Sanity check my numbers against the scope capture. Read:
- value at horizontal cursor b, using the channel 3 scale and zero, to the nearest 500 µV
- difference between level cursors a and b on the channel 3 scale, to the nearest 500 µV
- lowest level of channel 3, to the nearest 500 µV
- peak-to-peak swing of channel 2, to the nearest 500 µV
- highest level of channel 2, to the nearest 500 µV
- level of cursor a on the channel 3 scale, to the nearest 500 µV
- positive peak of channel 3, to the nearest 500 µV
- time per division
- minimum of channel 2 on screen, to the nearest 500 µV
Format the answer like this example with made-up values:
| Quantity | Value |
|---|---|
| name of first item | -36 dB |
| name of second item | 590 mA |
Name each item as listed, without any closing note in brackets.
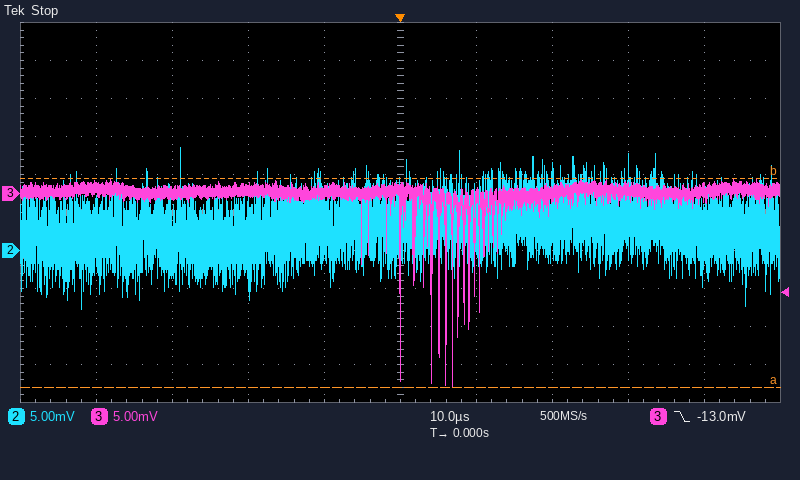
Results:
| Quantity | Value |
|---|---|
| value at horizontal cursor b, using the channel 3 scale and zero, to the nearest 500 µV | 2.0 mV |
| difference between level cursors a and b on the channel 3 scale, to the nearest 500 µV | 27.5 mV |
| lowest level of channel 3, to the nearest 500 µV | -25.5 mV |
| peak-to-peak swing of channel 2, to the nearest 500 µV | 21.0 mV |
| highest level of channel 2, to the nearest 500 µV | 13.5 mV |
| level of cursor a on the channel 3 scale, to the nearest 500 µV | -25.5 mV |
| positive peak of channel 3, to the nearest 500 µV | 2.0 mV |
| time per division | 10 µs |
| minimum of channel 2 on screen, to the nearest 500 µV | -7.5 mV |
